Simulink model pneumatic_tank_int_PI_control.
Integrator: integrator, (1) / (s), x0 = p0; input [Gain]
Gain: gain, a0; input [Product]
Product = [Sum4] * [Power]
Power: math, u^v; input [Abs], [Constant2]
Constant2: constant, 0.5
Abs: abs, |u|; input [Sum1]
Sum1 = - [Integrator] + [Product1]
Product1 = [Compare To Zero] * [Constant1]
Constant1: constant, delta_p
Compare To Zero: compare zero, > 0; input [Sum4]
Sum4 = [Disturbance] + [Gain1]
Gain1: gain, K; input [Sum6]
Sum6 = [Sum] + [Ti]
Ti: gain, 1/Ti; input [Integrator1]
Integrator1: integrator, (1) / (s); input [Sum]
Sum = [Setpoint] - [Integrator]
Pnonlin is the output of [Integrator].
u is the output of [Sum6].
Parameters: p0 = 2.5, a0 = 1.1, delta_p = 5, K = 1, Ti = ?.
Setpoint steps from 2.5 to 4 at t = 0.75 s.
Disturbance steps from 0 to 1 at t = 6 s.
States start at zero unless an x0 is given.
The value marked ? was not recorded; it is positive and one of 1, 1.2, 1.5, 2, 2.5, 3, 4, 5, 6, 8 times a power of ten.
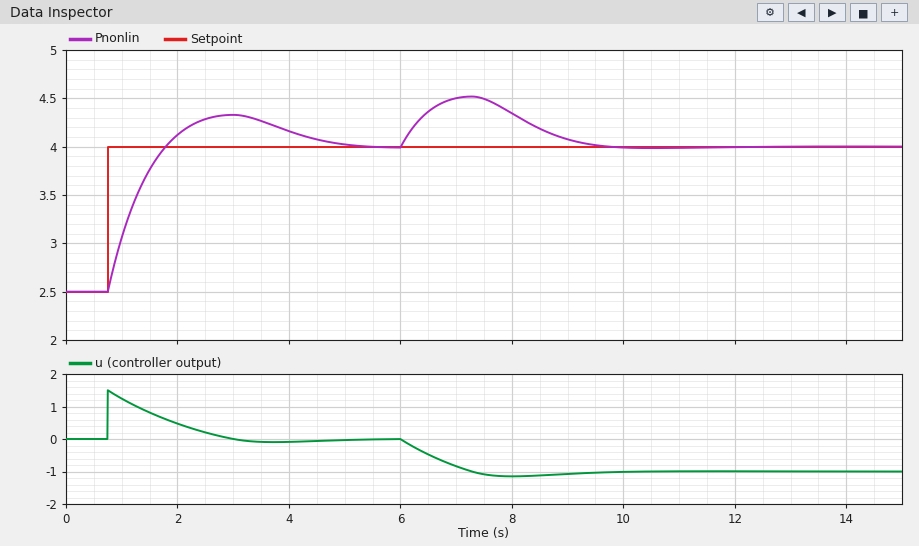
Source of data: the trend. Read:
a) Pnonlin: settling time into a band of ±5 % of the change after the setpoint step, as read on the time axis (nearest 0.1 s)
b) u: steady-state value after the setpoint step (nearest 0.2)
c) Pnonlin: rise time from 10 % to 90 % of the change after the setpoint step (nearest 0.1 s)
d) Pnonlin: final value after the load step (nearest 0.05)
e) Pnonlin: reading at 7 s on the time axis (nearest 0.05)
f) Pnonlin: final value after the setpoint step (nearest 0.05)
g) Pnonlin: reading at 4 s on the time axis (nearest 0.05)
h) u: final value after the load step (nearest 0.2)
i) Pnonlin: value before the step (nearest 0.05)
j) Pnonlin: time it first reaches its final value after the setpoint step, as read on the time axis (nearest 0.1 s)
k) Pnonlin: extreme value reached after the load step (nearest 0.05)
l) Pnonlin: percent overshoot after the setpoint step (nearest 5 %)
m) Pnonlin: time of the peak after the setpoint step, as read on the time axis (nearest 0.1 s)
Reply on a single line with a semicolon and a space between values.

4.5 s; 0.0; 0.8 s; 4.00; 4.50; 4.00; 4.15; -1.0; 2.50; 1.8 s; 4.50; 20 %; 3.0 s
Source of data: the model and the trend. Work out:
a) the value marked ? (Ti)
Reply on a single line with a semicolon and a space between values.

1
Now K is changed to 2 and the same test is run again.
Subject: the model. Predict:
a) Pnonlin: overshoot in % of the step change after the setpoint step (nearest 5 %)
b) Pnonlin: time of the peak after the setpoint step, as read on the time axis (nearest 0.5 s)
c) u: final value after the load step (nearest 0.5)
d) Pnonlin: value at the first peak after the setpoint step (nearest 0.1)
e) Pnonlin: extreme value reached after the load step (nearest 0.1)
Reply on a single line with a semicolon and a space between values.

15 %; 2.0 s; -0.5; 4.2; 4.3
